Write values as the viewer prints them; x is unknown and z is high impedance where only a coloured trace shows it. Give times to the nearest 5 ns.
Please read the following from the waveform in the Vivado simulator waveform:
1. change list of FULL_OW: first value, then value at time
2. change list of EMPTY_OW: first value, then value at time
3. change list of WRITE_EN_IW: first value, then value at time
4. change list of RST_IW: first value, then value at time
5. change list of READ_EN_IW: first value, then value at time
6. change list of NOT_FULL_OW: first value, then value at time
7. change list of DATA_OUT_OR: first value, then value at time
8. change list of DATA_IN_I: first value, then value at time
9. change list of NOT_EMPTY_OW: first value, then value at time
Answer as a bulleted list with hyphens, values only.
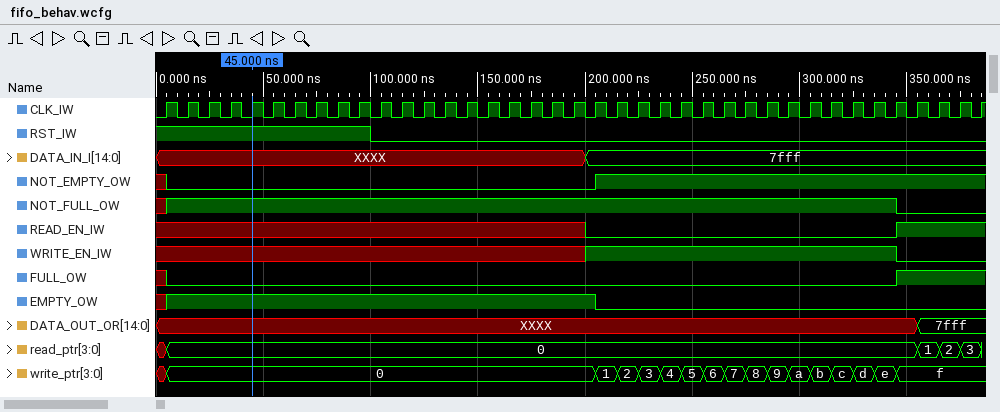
- x, 0 at 5 ns, 1 at 345 ns
- x, 1 at 5 ns, 0 at 205 ns
- x, 1 at 200 ns, 0 at 345 ns
- 1, 0 at 100 ns
- x, 0 at 200 ns, 1 at 345 ns
- x, 1 at 5 ns, 0 at 345 ns
- XXXX, 7fff at 355 ns
- XXXX, 7fff at 200 ns
- x, 0 at 5 ns, 1 at 205 ns
